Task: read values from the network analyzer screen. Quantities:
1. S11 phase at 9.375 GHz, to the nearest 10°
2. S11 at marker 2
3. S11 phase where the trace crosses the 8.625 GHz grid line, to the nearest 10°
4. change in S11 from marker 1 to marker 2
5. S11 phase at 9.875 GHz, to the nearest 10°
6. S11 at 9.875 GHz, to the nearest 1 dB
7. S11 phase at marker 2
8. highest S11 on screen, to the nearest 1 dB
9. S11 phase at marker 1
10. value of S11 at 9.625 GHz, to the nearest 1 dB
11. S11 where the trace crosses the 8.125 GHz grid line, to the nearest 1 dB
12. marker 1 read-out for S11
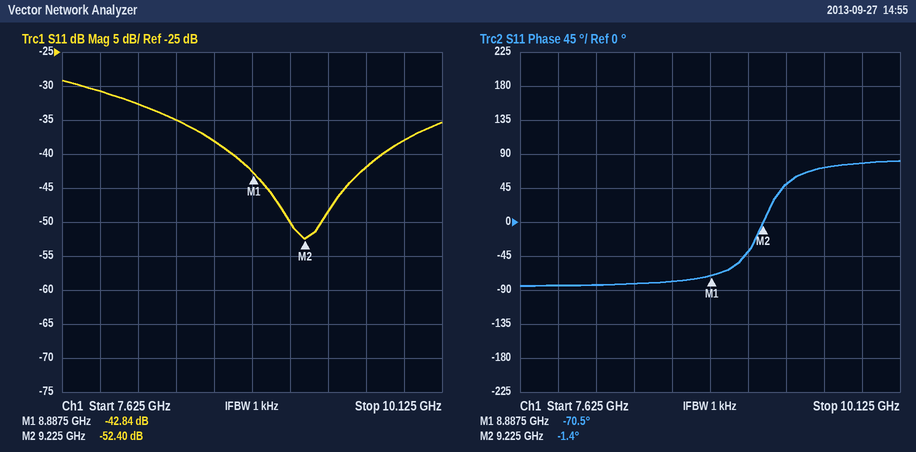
50°
-52.40 dB
-80°
-9.56 dB
80°
-38 dB
-1.4°
-29 dB
-70.5°
-42 dB
-33 dB
-42.84 dB
